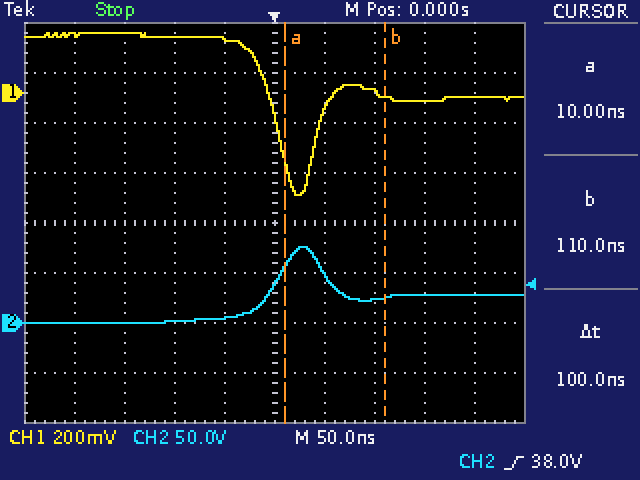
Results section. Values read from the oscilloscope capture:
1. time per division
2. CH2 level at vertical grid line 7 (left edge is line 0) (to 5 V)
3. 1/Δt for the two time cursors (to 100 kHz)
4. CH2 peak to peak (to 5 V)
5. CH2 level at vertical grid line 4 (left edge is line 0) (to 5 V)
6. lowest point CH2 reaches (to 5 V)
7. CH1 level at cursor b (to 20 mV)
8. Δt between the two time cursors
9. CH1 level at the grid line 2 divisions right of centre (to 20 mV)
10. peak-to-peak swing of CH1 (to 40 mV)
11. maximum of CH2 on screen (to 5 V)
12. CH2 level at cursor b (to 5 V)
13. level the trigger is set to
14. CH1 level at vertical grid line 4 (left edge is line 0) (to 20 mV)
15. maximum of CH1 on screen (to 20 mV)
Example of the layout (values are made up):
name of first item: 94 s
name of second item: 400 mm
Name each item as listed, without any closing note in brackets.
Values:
time per division: 50 ns
CH2 level at vertical grid line 7 (left edge is line 0): 25 V
1/Δt for the two time cursors: 10.0 MHz
CH2 peak to peak: 75 V
CH2 level at vertical grid line 4 (left edge is line 0): 5 V
lowest point CH2 reaches: 0 V
CH1 level at cursor b: -20 mV
Δt between the two time cursors: 100 ns
CH1 level at the grid line 2 divisions right of centre: 0 mV
peak-to-peak swing of CH1: 640 mV
maximum of CH2 on screen: 75 V
CH2 level at cursor b: 25 V
level the trigger is set to: 38.0 V
CH1 level at vertical grid line 4 (left edge is line 0): 220 mV
maximum of CH1 on screen: 240 mV
